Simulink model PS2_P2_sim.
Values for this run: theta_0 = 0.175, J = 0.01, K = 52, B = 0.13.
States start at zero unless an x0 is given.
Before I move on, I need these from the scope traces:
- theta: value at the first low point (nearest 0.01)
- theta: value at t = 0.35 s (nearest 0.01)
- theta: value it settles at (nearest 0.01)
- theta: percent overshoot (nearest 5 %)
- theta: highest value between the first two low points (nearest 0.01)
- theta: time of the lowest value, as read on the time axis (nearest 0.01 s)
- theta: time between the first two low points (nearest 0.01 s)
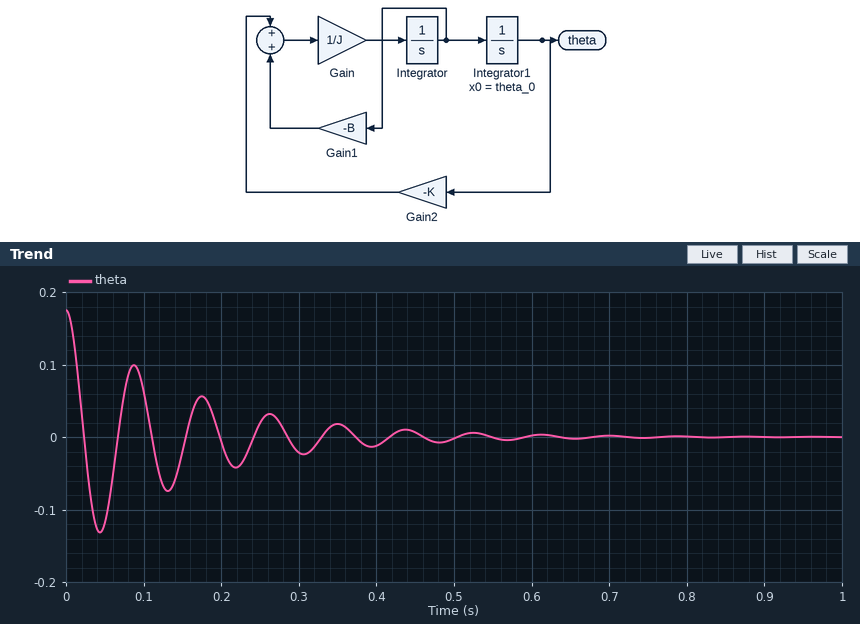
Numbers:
-0.13
0.02
0.00
75 %
0.10
0.04 s
0.09 s
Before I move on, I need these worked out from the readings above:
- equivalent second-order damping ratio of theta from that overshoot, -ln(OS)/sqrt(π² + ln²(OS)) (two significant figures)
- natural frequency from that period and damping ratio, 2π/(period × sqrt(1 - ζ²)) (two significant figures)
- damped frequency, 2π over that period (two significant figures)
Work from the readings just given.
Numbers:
0.091
70 rad/s
70 rad/s
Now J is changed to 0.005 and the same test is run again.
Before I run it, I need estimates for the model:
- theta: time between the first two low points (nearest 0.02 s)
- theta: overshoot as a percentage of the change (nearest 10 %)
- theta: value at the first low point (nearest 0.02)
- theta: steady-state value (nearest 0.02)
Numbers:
0.06 s
70 %
-0.12
0.00
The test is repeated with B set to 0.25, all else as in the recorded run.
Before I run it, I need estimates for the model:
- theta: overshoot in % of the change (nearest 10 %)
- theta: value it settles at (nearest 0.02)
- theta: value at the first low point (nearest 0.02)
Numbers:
60 %
0.00
-0.10
